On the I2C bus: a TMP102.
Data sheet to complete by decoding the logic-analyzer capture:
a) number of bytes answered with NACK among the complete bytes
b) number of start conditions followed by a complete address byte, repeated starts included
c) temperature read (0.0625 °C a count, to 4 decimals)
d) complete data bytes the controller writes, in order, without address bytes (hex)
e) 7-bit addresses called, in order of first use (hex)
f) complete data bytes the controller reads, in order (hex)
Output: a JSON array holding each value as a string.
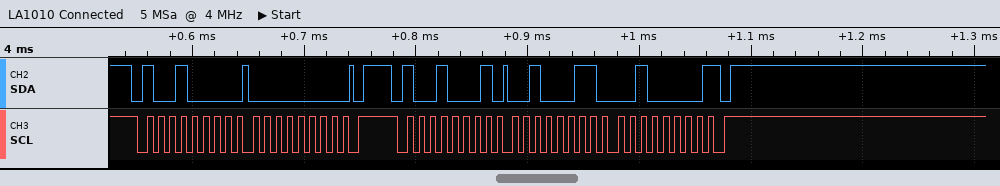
["1", "2", "35.1250 °C", "00", "0x48", "23 20"]
